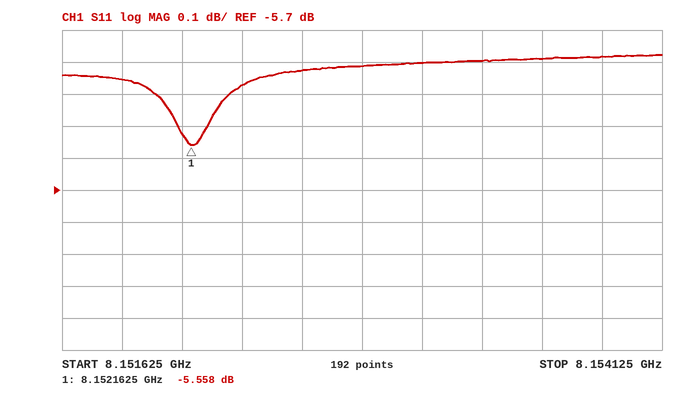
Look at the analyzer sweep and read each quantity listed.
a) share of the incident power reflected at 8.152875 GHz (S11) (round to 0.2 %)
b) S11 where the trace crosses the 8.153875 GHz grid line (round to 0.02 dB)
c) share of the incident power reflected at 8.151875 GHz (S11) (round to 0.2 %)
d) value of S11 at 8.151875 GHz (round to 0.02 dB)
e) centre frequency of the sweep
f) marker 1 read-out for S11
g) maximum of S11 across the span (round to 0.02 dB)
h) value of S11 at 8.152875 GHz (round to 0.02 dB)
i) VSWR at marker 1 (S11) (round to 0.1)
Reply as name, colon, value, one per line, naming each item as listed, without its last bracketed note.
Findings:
share of the incident power reflected at 8.152875 GHz (S11): 29.4 %
S11 where the trace crosses the 8.153875 GHz grid line: -5.28 dB
share of the incident power reflected at 8.151875 GHz (S11): 29.2 %
value of S11 at 8.151875 GHz: -5.36 dB
centre frequency of the sweep: 8.152875 GHz
marker 1 read-out for S11: -5.558 dB
maximum of S11 across the span: -5.28 dB
value of S11 at 8.152875 GHz: -5.32 dB
VSWR at marker 1 (S11): 3.2
